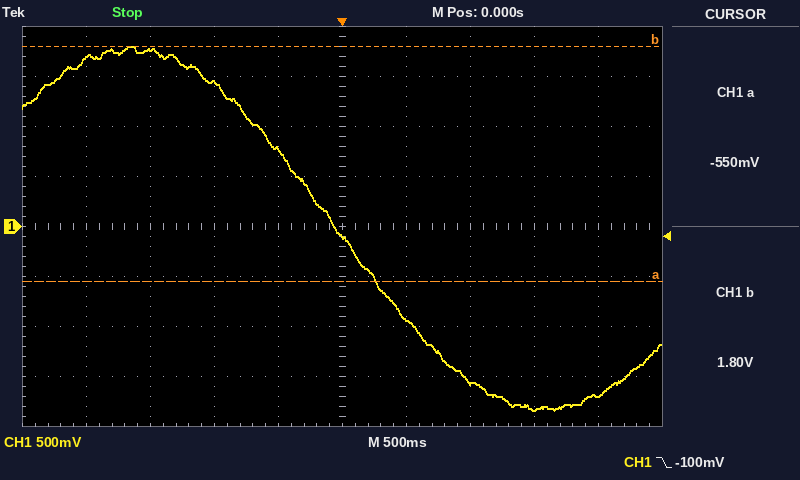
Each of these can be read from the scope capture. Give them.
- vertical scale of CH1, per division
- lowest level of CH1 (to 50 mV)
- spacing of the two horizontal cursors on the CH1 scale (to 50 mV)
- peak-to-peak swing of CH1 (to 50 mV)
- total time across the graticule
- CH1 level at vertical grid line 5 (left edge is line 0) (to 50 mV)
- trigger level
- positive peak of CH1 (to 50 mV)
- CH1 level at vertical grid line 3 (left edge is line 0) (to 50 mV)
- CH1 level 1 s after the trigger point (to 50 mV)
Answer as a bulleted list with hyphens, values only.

- 500 mV
- -1.85 V
- 2.35 V
- 3.65 V
- 5 s
- -100 mV
- -100 mV
- 1.80 V
- 1.45 V
- -1.55 V
